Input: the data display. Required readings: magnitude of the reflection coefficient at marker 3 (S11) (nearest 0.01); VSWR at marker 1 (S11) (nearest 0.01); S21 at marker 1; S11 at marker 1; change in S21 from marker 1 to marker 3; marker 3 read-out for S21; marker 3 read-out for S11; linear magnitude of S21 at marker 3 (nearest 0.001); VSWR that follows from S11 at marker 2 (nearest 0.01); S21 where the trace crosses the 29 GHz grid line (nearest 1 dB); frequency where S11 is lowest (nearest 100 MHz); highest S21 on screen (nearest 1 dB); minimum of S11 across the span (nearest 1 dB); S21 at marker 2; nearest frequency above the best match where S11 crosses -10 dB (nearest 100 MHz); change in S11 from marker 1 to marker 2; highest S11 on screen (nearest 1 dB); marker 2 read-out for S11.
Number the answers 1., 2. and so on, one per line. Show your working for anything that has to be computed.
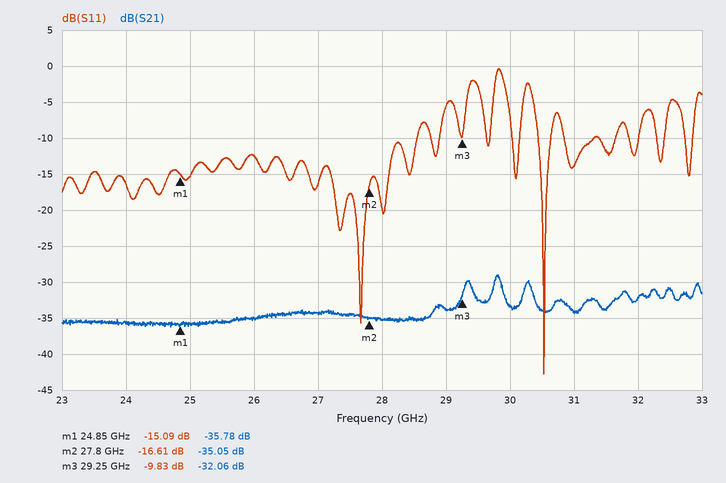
1. 10^(-9.83/20) ≈ 0.32
2. (1 + 0.1760)/(1 − 0.1760) ≈ 1.43
3. -35.78 dB
4. -15.09 dB
5. -32.06 − (-35.78) = 3.72 dB
6. -32.06 dB
7. -9.83 dB
8. 10^(-32.06/20) ≈ 0.025
9. (1 + 0.1477)/(1 − 0.1477) ≈ 1.35
10. -34 dB
11. 30.5 GHz
12. -29 dB
13. -43 dB
14. -35.05 dB
15. 30.6 GHz
16. -16.61 − (-15.09) = -1.52 dB
17. 0 dB
18. -16.61 dB
